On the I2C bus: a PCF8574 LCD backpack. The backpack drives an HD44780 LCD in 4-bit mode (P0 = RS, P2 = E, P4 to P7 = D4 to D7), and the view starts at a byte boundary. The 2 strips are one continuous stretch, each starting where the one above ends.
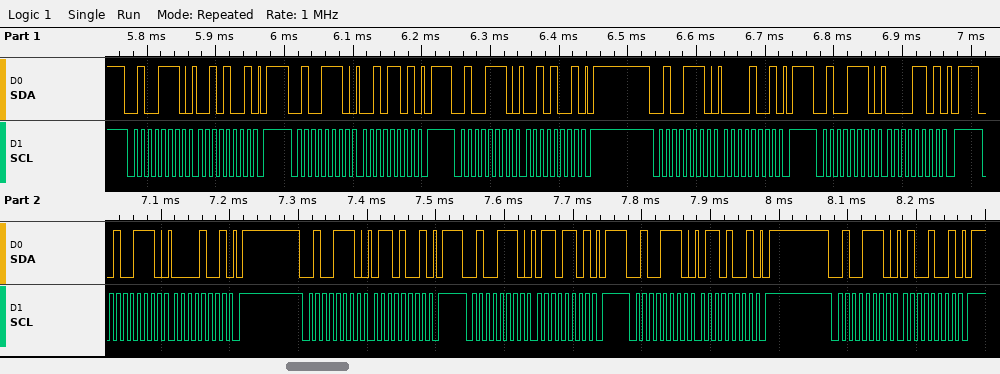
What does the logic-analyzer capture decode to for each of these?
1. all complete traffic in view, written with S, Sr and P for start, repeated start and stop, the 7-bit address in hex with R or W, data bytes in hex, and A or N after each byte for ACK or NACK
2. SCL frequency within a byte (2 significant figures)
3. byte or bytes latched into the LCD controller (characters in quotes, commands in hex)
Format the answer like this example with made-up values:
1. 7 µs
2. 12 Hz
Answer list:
1. S 27W A 29 A P S 27W A 2D A P S 27W A 29 A P S 27W A 09 A P S 27W A 0D A P S 27W A 09 A P S 27W A 69 A P S 27W A 6D A P S 27W A 69 A P S 27W A 49 A P
2. 100 kHz
3. ' '
